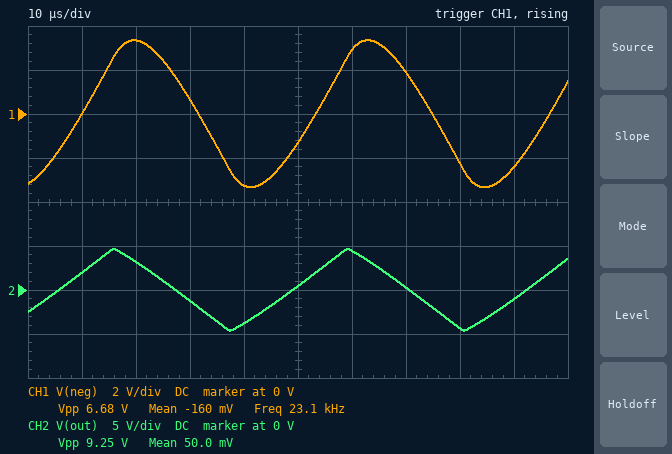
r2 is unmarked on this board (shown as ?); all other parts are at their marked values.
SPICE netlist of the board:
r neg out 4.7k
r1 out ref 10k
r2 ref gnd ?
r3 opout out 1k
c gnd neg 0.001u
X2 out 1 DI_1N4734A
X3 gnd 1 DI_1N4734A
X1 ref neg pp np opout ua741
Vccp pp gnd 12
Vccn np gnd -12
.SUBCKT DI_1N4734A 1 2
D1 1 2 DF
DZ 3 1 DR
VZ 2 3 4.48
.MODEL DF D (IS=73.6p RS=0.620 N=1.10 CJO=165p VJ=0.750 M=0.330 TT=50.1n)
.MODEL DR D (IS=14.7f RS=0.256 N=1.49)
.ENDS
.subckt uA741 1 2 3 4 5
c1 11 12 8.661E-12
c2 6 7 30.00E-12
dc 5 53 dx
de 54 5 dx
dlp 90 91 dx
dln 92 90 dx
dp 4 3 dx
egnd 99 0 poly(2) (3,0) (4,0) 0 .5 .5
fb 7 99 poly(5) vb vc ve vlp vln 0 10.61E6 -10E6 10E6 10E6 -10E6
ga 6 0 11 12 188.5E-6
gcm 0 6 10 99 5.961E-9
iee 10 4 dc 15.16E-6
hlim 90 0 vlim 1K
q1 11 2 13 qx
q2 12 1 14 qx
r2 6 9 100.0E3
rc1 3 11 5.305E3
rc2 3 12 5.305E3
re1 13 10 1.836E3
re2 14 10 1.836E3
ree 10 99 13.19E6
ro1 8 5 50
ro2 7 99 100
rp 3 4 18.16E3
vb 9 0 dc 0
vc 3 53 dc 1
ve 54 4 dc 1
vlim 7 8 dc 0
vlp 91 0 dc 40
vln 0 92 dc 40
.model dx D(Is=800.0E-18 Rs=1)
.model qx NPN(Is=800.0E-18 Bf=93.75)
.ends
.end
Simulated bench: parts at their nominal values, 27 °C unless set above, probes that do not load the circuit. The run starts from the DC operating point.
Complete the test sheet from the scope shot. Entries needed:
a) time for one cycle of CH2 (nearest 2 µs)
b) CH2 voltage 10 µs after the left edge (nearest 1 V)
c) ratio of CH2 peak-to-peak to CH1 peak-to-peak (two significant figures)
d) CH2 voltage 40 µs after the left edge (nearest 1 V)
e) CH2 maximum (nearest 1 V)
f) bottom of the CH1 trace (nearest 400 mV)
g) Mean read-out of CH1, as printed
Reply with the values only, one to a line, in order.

44 µs
2 V
1.4
-4 V
5 V
-3.2 V
-160 mV
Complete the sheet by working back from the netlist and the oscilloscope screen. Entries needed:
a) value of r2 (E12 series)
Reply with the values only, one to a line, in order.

12 kΩ
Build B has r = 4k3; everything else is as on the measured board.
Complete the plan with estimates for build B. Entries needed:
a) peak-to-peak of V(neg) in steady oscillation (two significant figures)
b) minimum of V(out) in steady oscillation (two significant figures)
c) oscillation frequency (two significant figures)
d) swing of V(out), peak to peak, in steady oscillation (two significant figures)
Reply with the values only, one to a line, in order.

6.1 V
-4.2 V
25 kHz
8.5 V
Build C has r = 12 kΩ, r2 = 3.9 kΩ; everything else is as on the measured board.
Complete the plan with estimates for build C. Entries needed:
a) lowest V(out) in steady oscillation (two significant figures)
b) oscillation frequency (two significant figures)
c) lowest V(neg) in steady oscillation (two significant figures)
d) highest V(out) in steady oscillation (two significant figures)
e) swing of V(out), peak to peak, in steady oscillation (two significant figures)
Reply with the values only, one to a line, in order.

-5.8 V
18 kHz
-2.9 V
5.8 V
12 V
